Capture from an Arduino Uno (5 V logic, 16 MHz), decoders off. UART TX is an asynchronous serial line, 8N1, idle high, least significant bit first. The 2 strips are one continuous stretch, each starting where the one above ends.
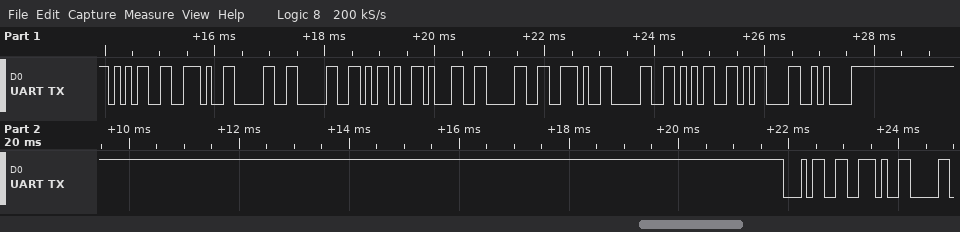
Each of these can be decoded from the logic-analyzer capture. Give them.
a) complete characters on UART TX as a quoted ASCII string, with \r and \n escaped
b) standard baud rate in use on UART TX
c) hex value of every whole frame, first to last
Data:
"5.00-10.05\r\n4."
9600 baud
0x35 0x2E 0x30 0x30 0x2D 0x31 0x30 0x2E 0x30 0x35 0x0D 0x0A 0x34 0x2E
